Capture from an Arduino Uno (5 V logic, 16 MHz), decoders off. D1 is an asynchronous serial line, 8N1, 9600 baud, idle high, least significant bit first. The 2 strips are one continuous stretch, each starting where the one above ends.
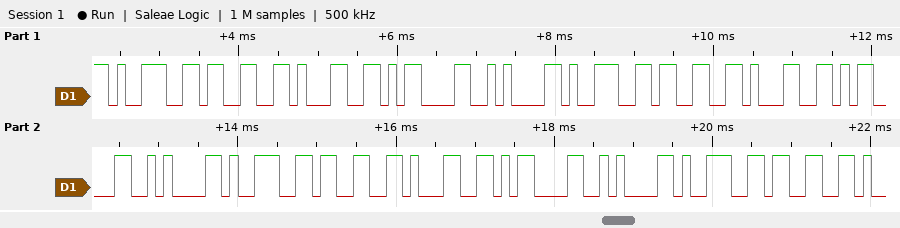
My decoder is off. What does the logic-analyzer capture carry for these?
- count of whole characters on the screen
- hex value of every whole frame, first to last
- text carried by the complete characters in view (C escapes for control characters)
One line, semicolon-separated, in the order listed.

17; 0x39 0x33 0x31 0x0D 0x0A 0x39 0x33 0x31 0x0D 0x0A 0x39 0x33 0x31 0x0D 0x0A 0x39 0x33; "931\r\n931\r\n931\r\n93"
